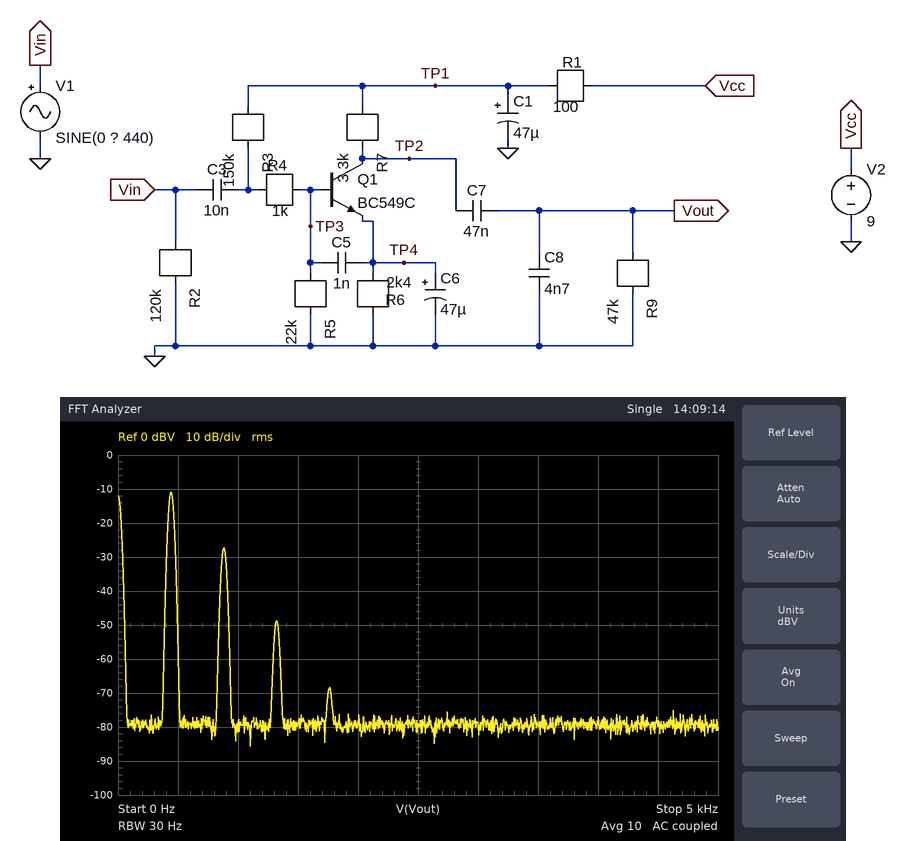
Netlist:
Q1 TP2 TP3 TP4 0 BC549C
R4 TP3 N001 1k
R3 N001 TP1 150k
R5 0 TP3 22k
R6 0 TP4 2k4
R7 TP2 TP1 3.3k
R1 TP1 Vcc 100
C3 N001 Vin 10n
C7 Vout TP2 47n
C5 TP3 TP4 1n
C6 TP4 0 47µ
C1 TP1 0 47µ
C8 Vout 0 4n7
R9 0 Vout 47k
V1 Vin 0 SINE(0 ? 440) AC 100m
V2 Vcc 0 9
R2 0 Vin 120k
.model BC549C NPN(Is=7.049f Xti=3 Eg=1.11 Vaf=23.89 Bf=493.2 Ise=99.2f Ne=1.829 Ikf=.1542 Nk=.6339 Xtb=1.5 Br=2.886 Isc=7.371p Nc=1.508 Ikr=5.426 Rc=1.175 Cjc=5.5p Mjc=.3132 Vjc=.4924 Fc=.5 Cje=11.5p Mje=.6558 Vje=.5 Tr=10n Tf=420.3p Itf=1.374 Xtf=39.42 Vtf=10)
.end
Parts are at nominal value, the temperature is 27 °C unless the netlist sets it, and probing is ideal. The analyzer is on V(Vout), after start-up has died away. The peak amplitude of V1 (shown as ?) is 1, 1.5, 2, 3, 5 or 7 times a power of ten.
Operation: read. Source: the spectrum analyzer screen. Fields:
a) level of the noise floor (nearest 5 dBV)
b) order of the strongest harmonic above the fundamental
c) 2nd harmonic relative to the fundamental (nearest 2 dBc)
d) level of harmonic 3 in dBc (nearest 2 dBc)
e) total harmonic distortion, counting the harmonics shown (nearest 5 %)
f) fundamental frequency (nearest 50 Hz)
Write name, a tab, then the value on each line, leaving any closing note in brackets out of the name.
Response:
level of the noise floor	-80 dBV
order of the strongest harmonic above the fundamental	2
2nd harmonic relative to the fundamental	-16 dBc
level of harmonic 3 in dBc	-38 dBc
total harmonic distortion, counting the harmonics shown	15 %
fundamental frequency	450 Hz
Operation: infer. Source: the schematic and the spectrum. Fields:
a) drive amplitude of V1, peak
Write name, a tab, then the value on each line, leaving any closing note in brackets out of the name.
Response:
drive amplitude of V1, peak	50 mV
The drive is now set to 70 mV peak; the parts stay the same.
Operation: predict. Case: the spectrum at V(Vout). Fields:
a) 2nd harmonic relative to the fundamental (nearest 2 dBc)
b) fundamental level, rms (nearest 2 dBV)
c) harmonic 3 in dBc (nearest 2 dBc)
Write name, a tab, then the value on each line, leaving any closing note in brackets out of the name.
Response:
2nd harmonic relative to the fundamental	-14 dBc
fundamental level, rms	-8 dBV
harmonic 3 in dBc	-32 dBc
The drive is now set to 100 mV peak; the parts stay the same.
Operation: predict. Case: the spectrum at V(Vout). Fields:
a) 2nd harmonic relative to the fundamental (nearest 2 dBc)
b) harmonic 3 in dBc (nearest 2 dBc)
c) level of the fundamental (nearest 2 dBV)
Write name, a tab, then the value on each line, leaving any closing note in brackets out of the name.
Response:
2nd harmonic relative to the fundamental	-10 dBc
harmonic 3 in dBc	-26 dBc
level of the fundamental	-6 dBV
